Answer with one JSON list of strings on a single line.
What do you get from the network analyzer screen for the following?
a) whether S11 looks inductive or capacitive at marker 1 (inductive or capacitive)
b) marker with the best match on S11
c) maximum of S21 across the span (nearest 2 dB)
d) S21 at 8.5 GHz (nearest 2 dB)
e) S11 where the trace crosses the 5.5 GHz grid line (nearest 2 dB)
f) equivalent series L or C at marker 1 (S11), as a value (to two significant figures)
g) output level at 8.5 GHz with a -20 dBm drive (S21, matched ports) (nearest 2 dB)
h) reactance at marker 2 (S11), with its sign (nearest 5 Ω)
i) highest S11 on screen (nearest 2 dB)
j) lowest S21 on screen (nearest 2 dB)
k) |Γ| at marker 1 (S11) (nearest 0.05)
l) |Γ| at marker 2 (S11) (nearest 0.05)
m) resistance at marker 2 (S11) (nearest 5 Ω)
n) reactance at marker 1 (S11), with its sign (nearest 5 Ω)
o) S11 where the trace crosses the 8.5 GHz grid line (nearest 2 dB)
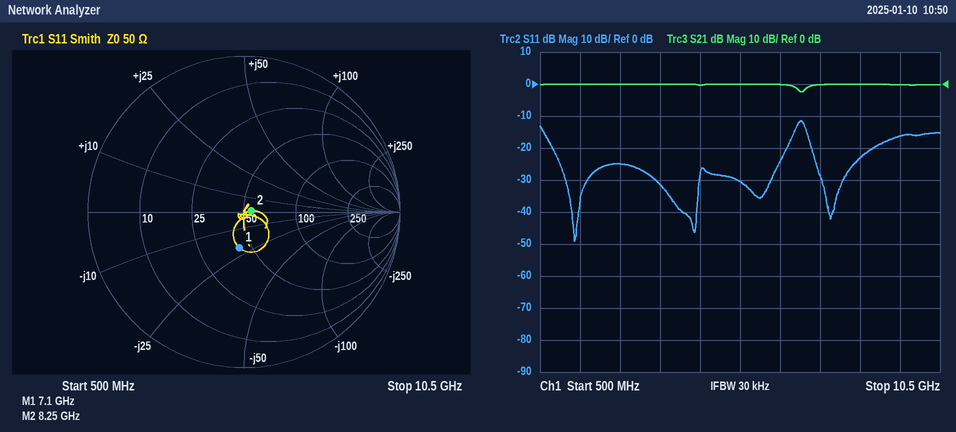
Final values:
["capacitive", "marker 2", "0 dB", "0 dB", "-30 dB", "1.1 pF", "-20 dBm", "0 Ω", "-12 dB", "-2 dB", "0.25", "0.05", "55 Ω", "-20 Ω", "-24 dB"]
